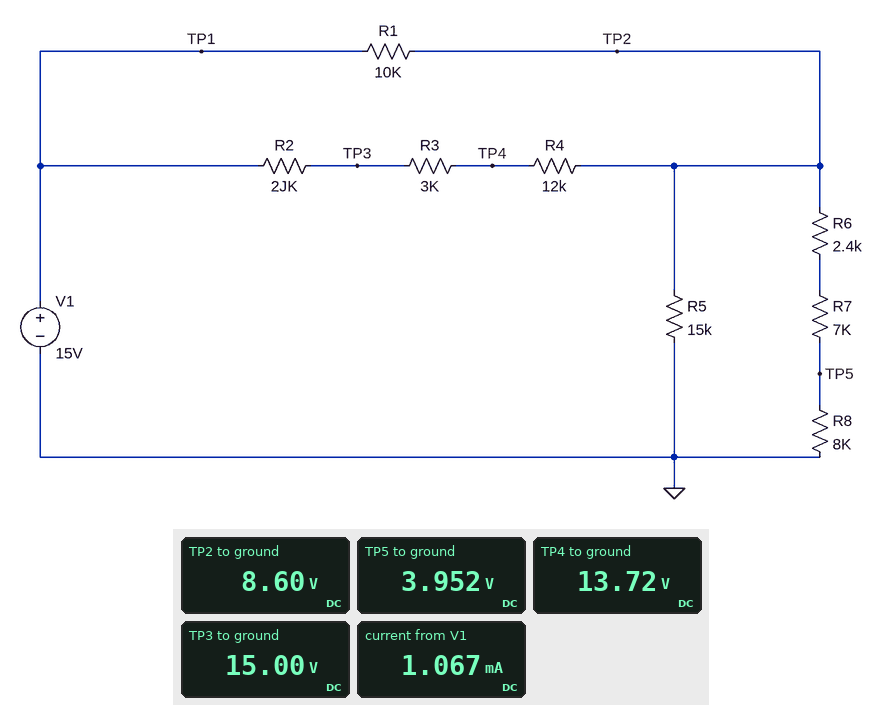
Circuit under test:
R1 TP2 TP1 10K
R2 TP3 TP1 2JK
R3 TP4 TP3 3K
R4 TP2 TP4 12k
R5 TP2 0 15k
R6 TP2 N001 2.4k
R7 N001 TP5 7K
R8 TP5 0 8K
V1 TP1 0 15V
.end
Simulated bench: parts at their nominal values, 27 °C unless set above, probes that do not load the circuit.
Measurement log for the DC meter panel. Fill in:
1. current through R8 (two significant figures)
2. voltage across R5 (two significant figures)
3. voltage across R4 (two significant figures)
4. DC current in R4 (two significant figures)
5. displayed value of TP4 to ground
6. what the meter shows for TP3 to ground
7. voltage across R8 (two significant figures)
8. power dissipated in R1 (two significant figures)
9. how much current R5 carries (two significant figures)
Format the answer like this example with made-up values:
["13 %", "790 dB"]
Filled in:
["490 µA", "8.6 V", "5.1 V", "430 µA", "13.72 V", "15.00 V", "4.0 V", "4.1 mW", "570 µA"]
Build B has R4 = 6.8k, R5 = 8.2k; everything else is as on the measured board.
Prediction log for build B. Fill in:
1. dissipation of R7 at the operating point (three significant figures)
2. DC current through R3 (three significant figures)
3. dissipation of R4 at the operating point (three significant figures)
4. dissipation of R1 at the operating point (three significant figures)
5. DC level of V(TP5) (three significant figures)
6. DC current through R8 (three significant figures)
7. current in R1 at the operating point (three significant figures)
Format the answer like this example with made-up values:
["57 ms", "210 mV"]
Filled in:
["1.46 mW", "720 µA", "3.52 mW", "4.98 mW", "3.65 V", "457 µA", "706 µA"]
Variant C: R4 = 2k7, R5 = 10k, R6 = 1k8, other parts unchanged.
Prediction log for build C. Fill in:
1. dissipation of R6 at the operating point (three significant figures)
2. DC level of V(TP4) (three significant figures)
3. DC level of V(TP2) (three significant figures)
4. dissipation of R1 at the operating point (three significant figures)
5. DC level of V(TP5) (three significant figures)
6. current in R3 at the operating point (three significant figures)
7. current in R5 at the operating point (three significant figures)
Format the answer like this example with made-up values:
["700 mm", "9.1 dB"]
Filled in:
["575 µW", "12.1 V", "9.50 V", "3.03 mW", "4.52 V", "965 µA", "950 µA"]
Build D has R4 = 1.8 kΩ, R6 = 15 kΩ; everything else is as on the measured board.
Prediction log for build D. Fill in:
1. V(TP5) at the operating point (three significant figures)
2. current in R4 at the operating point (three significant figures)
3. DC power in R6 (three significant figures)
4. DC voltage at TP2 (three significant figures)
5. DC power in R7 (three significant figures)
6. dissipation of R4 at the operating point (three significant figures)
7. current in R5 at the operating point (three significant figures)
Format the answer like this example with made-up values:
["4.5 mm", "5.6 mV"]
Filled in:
["3.02 V", "765 µA", "2.14 mW", "11.3 V", "998 µW", "1.05 mW", "755 µA"]
